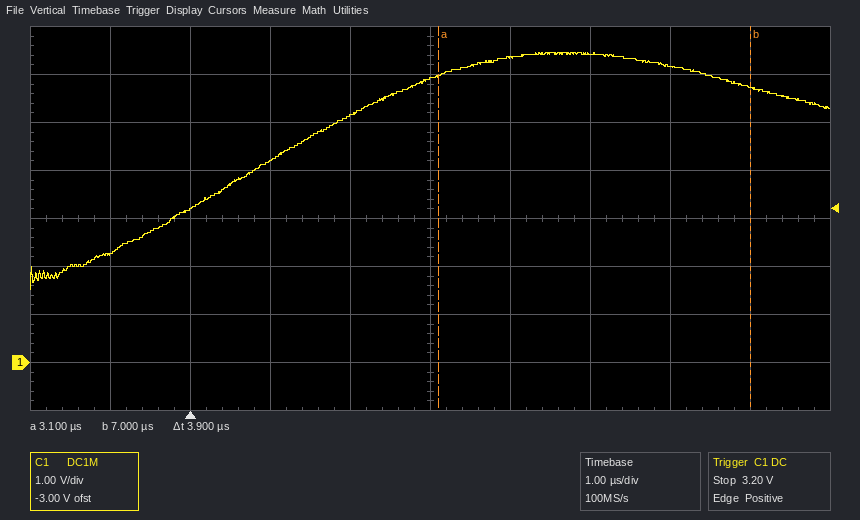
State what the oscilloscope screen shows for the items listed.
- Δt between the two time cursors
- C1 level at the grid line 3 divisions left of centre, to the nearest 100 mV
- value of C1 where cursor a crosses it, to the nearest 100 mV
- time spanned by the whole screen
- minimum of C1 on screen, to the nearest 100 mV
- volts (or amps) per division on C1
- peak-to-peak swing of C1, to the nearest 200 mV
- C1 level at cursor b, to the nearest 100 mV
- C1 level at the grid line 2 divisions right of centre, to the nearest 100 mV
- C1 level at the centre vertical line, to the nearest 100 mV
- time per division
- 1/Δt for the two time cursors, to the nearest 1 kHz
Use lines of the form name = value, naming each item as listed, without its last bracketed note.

Δt between the two time cursors = 3.9 µs
C1 level at the grid line 3 divisions left of centre, to the nearest 100 mV = 3.2 V
value of C1 where cursor a crosses it, to the nearest 100 mV = 6.0 V
time spanned by the whole screen = 10 µs
minimum of C1 on screen, to the nearest 100 mV = 1.5 V
volts (or amps) per division on C1 = 1 V
peak-to-peak swing of C1, to the nearest 200 mV = 5.0 V
C1 level at cursor b, to the nearest 100 mV = 5.7 V
C1 level at the grid line 2 divisions right of centre, to the nearest 100 mV = 6.4 V
C1 level at the centre vertical line, to the nearest 100 mV = 5.9 V
time per division = 1 µs
1/Δt for the two time cursors, to the nearest 1 kHz = 256 kHz
